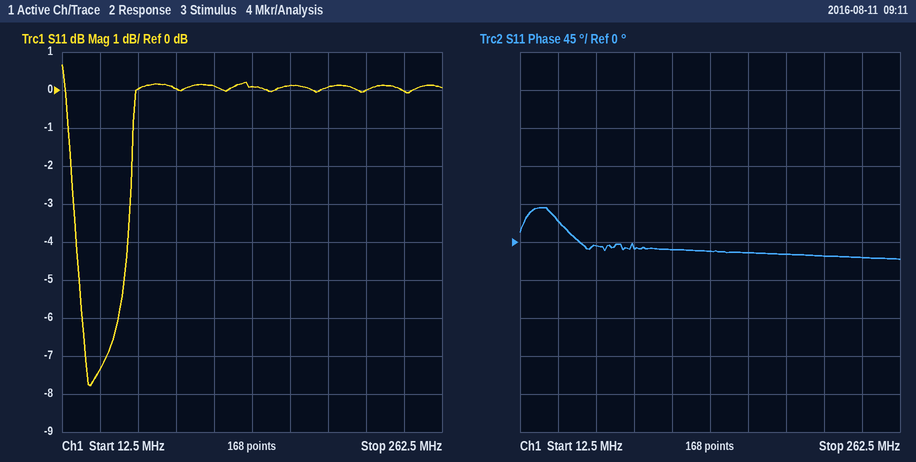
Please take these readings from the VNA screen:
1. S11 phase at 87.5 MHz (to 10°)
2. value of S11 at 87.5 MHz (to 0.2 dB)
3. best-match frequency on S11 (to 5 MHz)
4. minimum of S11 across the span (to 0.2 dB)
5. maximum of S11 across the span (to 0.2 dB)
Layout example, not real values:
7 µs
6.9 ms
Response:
-10°
0.0 dB
30 MHz
-7.8 dB
0.6 dB
